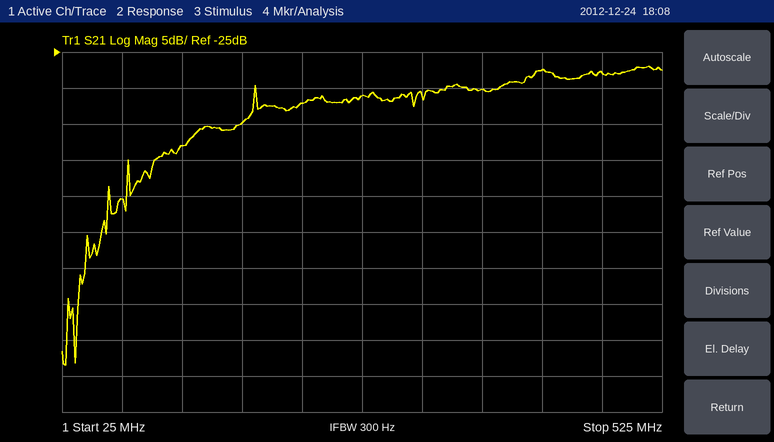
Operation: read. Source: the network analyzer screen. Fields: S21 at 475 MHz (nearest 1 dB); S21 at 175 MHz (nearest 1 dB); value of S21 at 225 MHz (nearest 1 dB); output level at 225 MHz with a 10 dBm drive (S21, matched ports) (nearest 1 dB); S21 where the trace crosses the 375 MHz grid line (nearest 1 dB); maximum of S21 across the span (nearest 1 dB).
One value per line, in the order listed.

-28 dB
-35 dB
-32 dB
-22 dBm
-30 dB
-27 dB
